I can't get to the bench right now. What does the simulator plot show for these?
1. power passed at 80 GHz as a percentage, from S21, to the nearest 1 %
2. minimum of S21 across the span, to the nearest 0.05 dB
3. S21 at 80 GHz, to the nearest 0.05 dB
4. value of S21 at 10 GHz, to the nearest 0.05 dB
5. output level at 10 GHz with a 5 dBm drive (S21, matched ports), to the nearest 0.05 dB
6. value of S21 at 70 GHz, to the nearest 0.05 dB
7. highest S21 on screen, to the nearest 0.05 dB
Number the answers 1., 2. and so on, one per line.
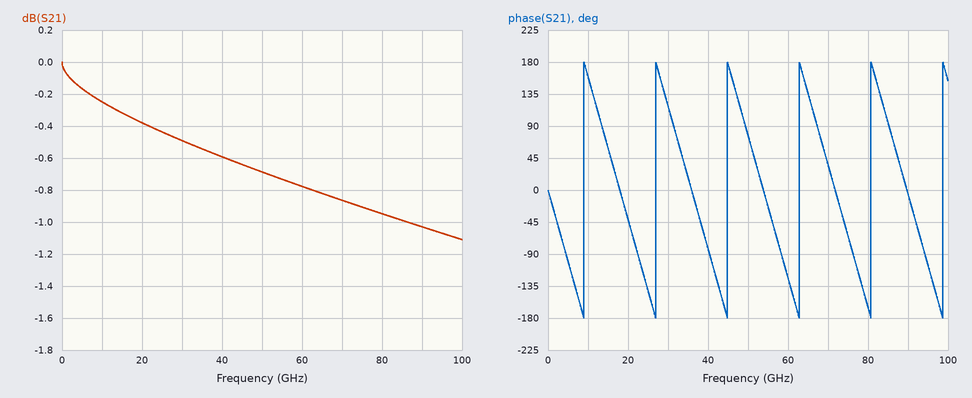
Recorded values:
1. 80 %
2. -1.10 dB
3. -0.95 dB
4. -0.25 dB
5. 4.75 dBm
6. -0.85 dB
7. 0.00 dB
